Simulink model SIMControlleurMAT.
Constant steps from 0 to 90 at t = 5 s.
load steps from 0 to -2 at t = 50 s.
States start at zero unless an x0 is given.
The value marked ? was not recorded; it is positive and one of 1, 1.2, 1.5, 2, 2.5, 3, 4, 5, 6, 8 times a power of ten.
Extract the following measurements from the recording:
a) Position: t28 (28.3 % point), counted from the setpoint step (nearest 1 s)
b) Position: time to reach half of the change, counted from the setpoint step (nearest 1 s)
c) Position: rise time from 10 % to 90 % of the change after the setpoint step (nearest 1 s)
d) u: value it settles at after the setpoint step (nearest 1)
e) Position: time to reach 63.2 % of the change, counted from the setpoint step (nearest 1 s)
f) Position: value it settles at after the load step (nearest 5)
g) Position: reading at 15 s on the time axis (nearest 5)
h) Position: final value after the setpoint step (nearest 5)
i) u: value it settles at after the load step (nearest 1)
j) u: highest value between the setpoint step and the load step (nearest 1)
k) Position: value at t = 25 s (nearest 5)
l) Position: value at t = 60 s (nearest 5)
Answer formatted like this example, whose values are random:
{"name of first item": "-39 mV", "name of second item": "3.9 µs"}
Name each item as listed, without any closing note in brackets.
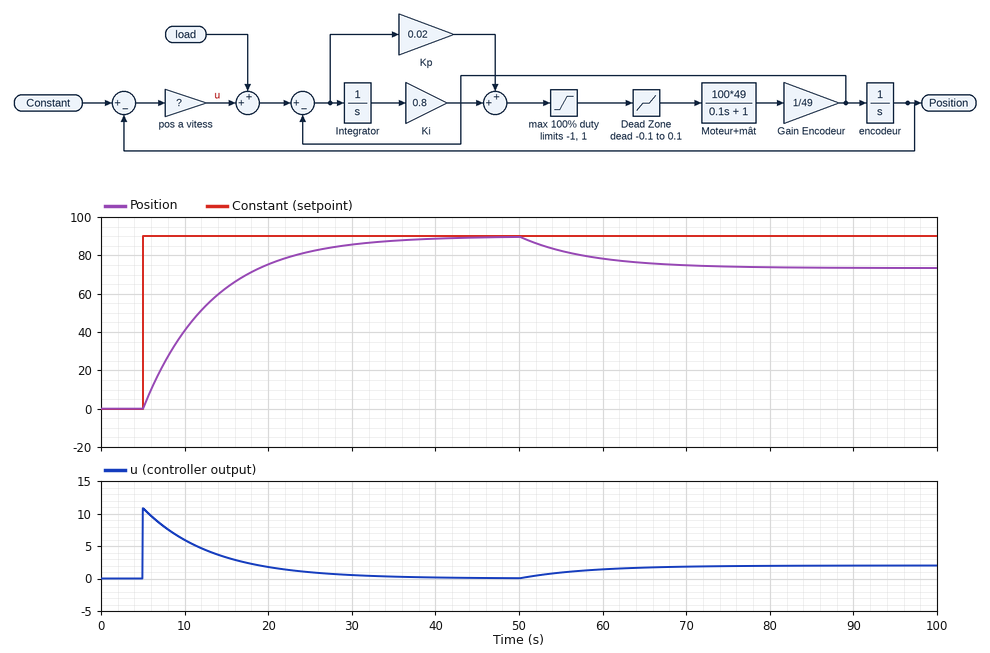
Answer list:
{"Position: t28 (28.3 % point), counted from the setpoint step": "3 s", "Position: time to reach half of the change, counted from the setpoint step": "6 s", "Position: rise time from 10 % to 90 % of the change after the setpoint step": "18 s", "u: value it settles at after the setpoint step": "0", "Position: time to reach 63.2 % of the change, counted from the setpoint step": "8 s", "Position: value it settles at after the load step": "75", "Position: reading at 15 s on the time axis": "65", "Position: final value after the setpoint step": "90", "u: value it settles at after the load step": "2", "u: highest value between the setpoint step and the load step": "11", "Position: value at t = 25 s": "80", "Position: value at t = 60 s": "80"}
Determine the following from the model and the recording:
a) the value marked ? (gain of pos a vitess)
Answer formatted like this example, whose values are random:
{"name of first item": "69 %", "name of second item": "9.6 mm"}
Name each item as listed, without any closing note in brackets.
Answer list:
{"the value marked ?": "0.12"}
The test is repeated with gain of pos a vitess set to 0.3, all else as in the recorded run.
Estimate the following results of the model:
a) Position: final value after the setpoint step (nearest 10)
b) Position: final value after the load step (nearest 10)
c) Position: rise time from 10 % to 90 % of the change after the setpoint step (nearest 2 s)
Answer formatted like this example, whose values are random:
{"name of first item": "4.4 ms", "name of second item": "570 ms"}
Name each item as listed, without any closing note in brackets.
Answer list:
{"Position: final value after the setpoint step": "90", "Position: final value after the load step": "80", "Position: rise time from 10 % to 90 % of the change after the setpoint step": "8 s"}
